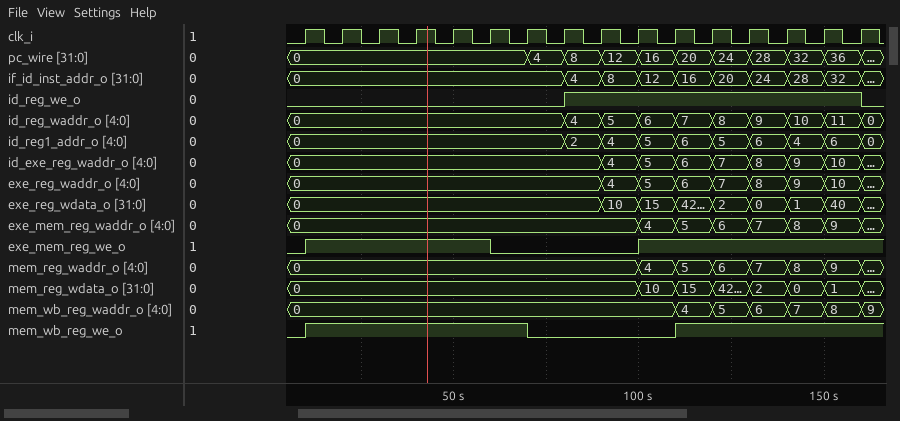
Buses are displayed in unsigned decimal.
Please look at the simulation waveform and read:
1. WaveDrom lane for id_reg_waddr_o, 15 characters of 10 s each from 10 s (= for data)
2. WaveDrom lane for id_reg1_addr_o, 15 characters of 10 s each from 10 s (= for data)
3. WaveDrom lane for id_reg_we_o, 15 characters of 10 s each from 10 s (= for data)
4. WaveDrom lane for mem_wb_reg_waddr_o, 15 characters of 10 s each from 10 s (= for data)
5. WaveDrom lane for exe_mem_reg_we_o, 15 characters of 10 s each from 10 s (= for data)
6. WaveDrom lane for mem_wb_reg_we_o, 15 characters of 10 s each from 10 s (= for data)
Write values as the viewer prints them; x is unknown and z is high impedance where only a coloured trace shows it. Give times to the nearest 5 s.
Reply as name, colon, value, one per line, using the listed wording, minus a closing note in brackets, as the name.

WaveDrom lane for id_reg_waddr_o, 15 characters of 10 s each from 10 s: {name: 'id_reg_waddr_o', wave: '=......========', data: '0 4 5 6 7 8 9 10 11'}
WaveDrom lane for id_reg1_addr_o, 15 characters of 10 s each from 10 s: {name: 'id_reg1_addr_o', wave: '=......========', data: '0 2 4 5 6 5 6 4 6'}
WaveDrom lane for id_reg_we_o, 15 characters of 10 s each from 10 s: {name: 'id_reg_we_o', wave: '0......1.......'}
WaveDrom lane for mem_wb_reg_waddr_o, 15 characters of 10 s each from 10 s: {name: 'mem_wb_reg_waddr_o', wave: '=.........=====', data: '0 4 5 6 7 8'}
WaveDrom lane for exe_mem_reg_we_o, 15 characters of 10 s each from 10 s: {name: 'exe_mem_reg_we_o', wave: '1....0...1.....'}
WaveDrom lane for mem_wb_reg_we_o, 15 characters of 10 s each from 10 s: {name: 'mem_wb_reg_we_o', wave: '1.....0...1....'}
